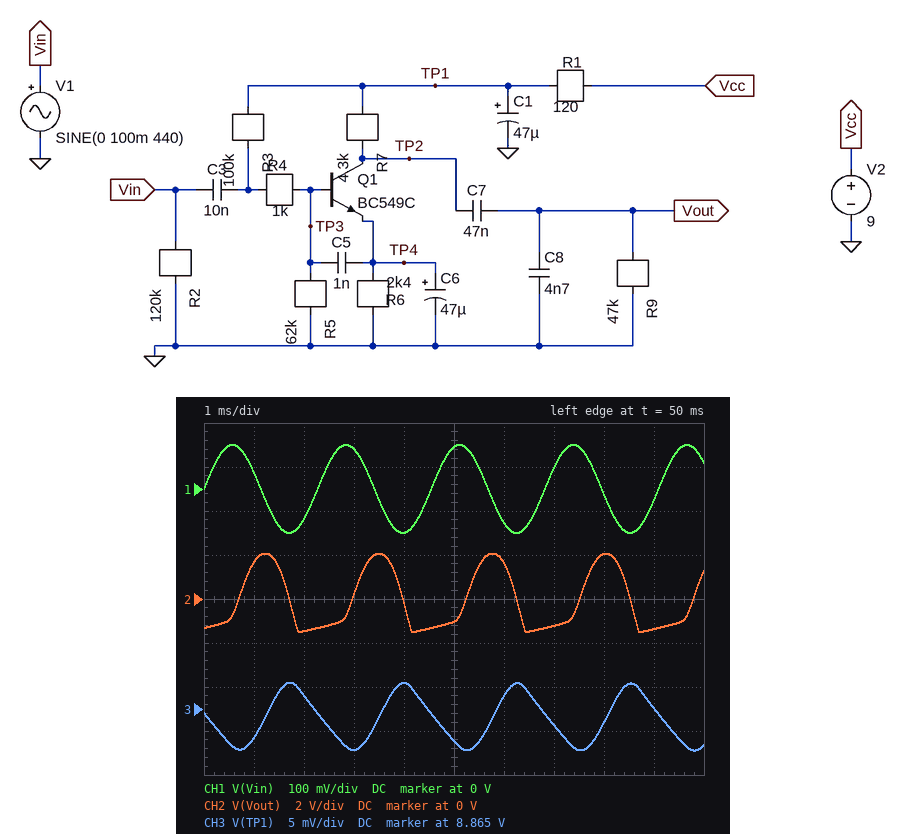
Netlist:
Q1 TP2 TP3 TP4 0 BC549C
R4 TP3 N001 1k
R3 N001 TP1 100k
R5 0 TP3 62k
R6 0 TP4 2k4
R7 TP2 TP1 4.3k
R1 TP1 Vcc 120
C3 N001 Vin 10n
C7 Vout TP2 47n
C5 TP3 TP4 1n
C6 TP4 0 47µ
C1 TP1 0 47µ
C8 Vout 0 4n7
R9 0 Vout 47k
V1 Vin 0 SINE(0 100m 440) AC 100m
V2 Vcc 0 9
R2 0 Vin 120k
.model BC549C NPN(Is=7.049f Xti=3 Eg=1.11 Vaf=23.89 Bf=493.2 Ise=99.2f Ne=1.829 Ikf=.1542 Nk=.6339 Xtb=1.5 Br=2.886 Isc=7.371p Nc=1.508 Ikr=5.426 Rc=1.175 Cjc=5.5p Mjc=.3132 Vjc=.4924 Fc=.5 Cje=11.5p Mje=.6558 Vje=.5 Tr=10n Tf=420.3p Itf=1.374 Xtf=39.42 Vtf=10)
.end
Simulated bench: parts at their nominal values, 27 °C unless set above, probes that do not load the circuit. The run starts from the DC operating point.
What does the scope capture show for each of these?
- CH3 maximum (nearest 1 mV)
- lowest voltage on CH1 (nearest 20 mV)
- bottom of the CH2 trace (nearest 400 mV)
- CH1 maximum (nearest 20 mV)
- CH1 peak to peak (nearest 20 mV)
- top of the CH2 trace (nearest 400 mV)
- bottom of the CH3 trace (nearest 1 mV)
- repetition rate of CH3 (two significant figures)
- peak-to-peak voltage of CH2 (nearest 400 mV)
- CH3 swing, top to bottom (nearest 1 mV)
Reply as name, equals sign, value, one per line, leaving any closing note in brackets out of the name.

CH3 maximum = 8.868 V
lowest voltage on CH1 = -100 mV
bottom of the CH2 trace = -1.6 V
CH1 maximum = 100 mV
CH1 peak to peak = 200 mV
top of the CH2 trace = 2.0 V
bottom of the CH3 trace = 8.860 V
repetition rate of CH3 = 440 Hz
peak-to-peak voltage of CH2 = 3.6 V
CH3 swing, top to bottom = 8 mV
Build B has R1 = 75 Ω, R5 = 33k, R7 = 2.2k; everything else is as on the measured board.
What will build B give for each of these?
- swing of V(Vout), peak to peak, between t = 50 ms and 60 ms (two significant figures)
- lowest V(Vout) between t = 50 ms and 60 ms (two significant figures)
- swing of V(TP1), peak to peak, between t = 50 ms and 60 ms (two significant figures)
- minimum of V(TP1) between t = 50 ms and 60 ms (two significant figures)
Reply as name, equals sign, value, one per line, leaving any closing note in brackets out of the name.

swing of V(Vout), peak to peak, between t = 50 ms and 60 ms = 2.4 V
lowest V(Vout) between t = 50 ms and 60 ms = -1.4 V
swing of V(TP1), peak to peak, between t = 50 ms and 60 ms = 9.4 mV
minimum of V(TP1) between t = 50 ms and 60 ms = 8.9 V
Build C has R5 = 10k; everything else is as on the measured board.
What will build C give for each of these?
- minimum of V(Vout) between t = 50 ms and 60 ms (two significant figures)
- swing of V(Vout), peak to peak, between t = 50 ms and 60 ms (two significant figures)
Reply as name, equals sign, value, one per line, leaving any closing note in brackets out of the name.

minimum of V(Vout) between t = 50 ms and 60 ms = -320 mV
swing of V(Vout), peak to peak, between t = 50 ms and 60 ms = 530 mV
